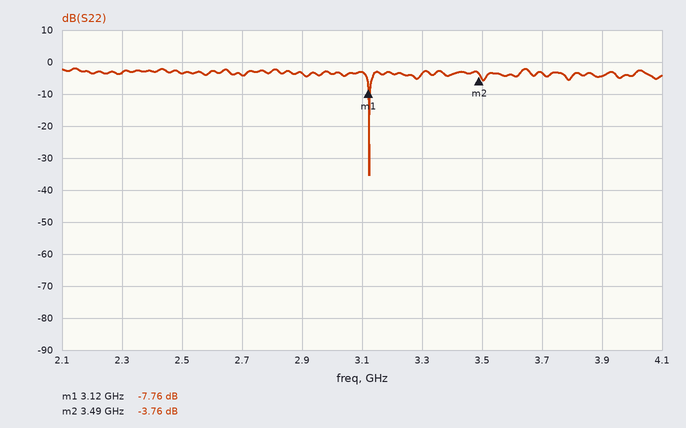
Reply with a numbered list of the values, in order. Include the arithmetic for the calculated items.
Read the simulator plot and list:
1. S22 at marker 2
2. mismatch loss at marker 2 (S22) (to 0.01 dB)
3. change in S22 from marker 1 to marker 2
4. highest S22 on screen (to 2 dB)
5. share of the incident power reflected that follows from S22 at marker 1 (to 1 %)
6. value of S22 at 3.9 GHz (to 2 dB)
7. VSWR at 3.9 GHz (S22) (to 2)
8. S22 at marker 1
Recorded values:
1. -3.76 dB
2. −10 log10(1 − 10^(-3.76/10)) ≈ 2.37 dB
3. -3.76 − (-7.76) = 4.00 dB
4. -2 dB
5. 10^(-7.76/10) ≈ 17 %
6. -4 dB
7. |Γ| = 10^(-4/20) = 0.6310; VSWR = (1 + 0.6310)/(1 − 0.6310) ≈ 4
8. -7.76 dB
